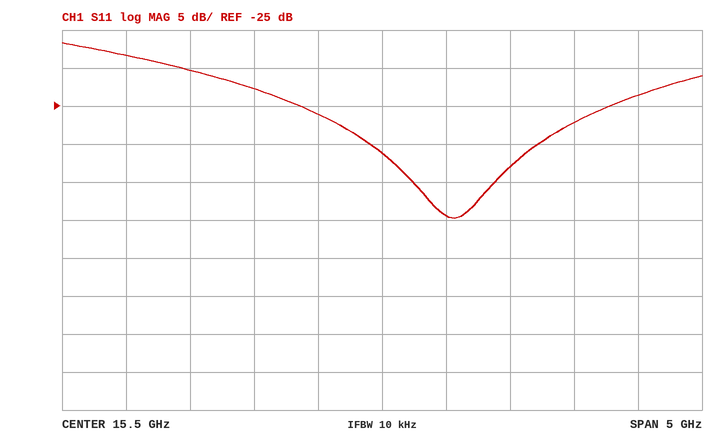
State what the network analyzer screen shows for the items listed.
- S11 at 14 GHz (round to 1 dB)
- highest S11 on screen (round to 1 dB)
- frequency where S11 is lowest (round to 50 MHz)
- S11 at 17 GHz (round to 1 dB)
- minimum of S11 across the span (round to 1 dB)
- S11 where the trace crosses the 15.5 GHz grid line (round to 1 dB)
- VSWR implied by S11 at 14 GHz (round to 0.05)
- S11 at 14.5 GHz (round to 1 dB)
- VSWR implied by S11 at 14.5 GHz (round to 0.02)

-20 dB
-17 dB
16.05 GHz
-27 dB
-40 dB
-31 dB
1.20
-23 dB
1.16
